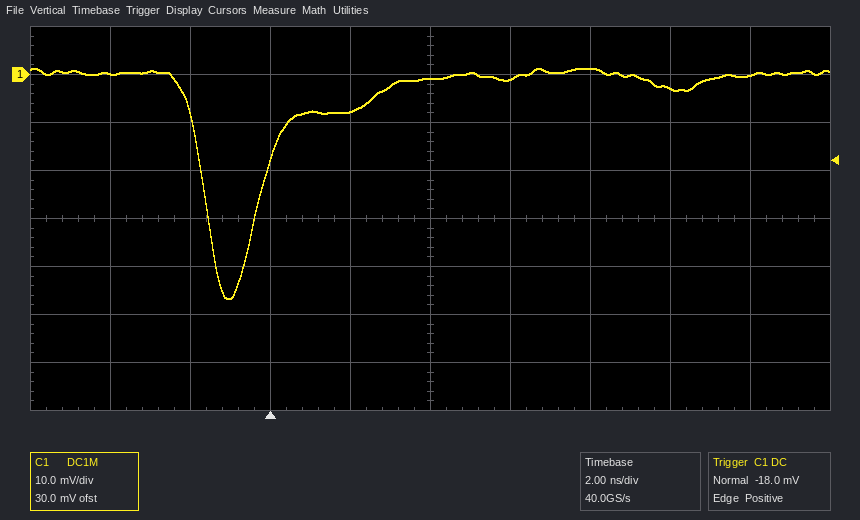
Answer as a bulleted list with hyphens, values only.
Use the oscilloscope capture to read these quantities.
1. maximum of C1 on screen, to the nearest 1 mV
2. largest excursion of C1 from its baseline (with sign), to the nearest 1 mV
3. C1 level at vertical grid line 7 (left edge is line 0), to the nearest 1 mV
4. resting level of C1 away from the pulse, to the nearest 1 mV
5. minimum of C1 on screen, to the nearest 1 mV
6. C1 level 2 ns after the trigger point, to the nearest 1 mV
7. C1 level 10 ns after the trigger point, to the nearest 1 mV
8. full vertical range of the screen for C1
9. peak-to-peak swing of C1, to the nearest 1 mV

- 1 mV
- -47 mV
- 1 mV
- 0 mV
- -47 mV
- -8 mV
- -3 mV
- 80 mV
- 48 mV
